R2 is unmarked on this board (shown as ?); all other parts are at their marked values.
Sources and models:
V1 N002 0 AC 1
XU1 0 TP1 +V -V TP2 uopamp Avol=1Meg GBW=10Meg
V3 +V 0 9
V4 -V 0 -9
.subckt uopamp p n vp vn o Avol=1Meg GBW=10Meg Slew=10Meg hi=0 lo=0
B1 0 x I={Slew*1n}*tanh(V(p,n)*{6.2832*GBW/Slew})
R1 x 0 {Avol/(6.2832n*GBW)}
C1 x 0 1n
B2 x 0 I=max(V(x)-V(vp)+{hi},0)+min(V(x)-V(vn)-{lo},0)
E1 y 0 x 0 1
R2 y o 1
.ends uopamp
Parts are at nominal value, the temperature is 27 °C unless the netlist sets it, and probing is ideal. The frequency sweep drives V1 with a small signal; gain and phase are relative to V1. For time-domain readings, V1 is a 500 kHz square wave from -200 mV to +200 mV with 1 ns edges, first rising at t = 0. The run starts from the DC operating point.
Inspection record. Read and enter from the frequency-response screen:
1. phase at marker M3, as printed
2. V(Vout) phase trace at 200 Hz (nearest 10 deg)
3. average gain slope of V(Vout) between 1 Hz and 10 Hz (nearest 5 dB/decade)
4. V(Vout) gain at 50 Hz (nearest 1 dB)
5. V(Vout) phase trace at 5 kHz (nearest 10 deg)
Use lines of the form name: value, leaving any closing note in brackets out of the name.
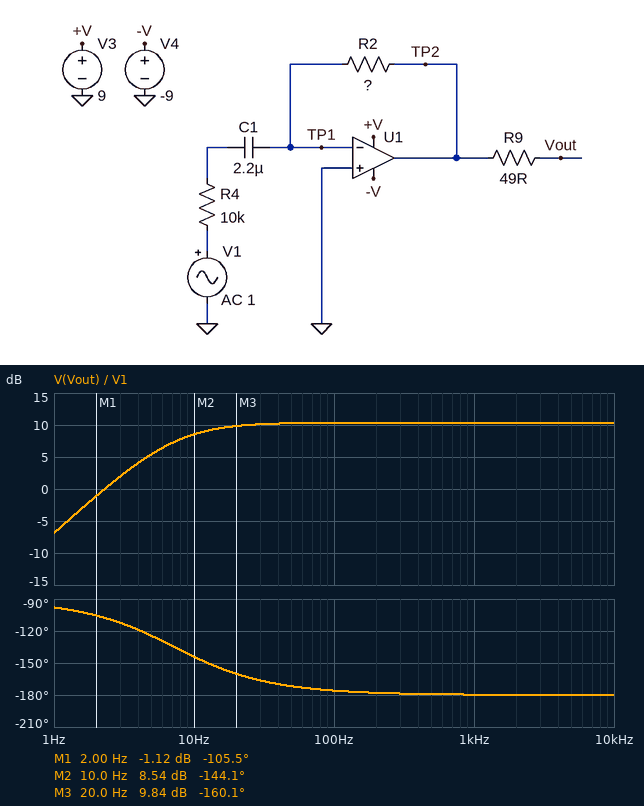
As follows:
phase at marker M3, as printed: -160.1 deg
V(Vout) phase trace at 200 Hz: -180 deg
average gain slope of V(Vout) between 1 Hz and 10 Hz: 15 dB/decade
V(Vout) gain at 50 Hz: 10 dB
V(Vout) phase trace at 5 kHz: -180 deg
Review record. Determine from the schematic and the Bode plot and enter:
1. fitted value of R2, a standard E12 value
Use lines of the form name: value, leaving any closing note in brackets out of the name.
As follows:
fitted value of R2, a standard E12 value: 33 kΩ
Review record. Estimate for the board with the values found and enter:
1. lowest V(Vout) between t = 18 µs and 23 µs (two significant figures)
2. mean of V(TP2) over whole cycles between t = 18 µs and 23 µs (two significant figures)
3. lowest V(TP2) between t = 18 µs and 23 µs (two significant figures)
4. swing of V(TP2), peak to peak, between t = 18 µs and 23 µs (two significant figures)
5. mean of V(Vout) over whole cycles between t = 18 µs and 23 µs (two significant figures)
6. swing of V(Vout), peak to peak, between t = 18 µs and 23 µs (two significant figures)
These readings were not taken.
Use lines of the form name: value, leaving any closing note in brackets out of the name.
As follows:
lowest V(Vout) between t = 18 µs and 23 µs: -1.3 V
mean of V(TP2) over whole cycles between t = 18 µs and 23 µs: -660 mV
lowest V(TP2) between t = 18 µs and 23 µs: -1.3 V
swing of V(TP2), peak to peak, between t = 18 µs and 23 µs: 1.3 V
mean of V(Vout) over whole cycles between t = 18 µs and 23 µs: -660 mV
swing of V(Vout), peak to peak, between t = 18 µs and 23 µs: 1.3 V
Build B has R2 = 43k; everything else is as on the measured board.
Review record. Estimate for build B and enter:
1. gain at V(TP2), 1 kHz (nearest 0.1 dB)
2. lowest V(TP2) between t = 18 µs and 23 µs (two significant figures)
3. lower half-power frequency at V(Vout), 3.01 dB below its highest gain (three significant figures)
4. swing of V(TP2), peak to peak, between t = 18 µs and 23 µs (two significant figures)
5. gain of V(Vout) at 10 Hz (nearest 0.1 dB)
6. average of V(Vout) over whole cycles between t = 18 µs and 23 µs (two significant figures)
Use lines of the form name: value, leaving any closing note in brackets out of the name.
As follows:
gain at V(TP2), 1 kHz: 12.7 dB
lowest V(TP2) between t = 18 µs and 23 µs: -1.7 V
lower half-power frequency at V(Vout), 3.01 dB below its highest gain: 7.23 Hz
swing of V(TP2), peak to peak, between t = 18 µs and 23 µs: 1.7 V
gain of V(Vout) at 10 Hz: 10.8 dB
average of V(Vout) over whole cycles between t = 18 µs and 23 µs: -860 mV
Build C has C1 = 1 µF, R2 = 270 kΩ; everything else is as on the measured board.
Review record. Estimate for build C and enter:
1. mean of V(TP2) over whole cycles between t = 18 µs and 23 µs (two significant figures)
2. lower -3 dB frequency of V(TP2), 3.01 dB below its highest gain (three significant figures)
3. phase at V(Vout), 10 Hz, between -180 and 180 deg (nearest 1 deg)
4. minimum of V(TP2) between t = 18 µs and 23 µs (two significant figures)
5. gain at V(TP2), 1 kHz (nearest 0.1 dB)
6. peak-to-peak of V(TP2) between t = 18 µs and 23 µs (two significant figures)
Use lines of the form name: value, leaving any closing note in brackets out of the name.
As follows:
mean of V(TP2) over whole cycles between t = 18 µs and 23 µs: -5.4 V
lower -3 dB frequency of V(TP2), 3.01 dB below its highest gain: 15.9 Hz
phase at V(Vout), 10 Hz, between -180 and 180 deg: -122 deg
minimum of V(TP2) between t = 18 µs and 23 µs: -9.0 V
gain at V(TP2), 1 kHz: 28.6 dB
peak-to-peak of V(TP2) between t = 18 µs and 23 µs: 7.3 V
